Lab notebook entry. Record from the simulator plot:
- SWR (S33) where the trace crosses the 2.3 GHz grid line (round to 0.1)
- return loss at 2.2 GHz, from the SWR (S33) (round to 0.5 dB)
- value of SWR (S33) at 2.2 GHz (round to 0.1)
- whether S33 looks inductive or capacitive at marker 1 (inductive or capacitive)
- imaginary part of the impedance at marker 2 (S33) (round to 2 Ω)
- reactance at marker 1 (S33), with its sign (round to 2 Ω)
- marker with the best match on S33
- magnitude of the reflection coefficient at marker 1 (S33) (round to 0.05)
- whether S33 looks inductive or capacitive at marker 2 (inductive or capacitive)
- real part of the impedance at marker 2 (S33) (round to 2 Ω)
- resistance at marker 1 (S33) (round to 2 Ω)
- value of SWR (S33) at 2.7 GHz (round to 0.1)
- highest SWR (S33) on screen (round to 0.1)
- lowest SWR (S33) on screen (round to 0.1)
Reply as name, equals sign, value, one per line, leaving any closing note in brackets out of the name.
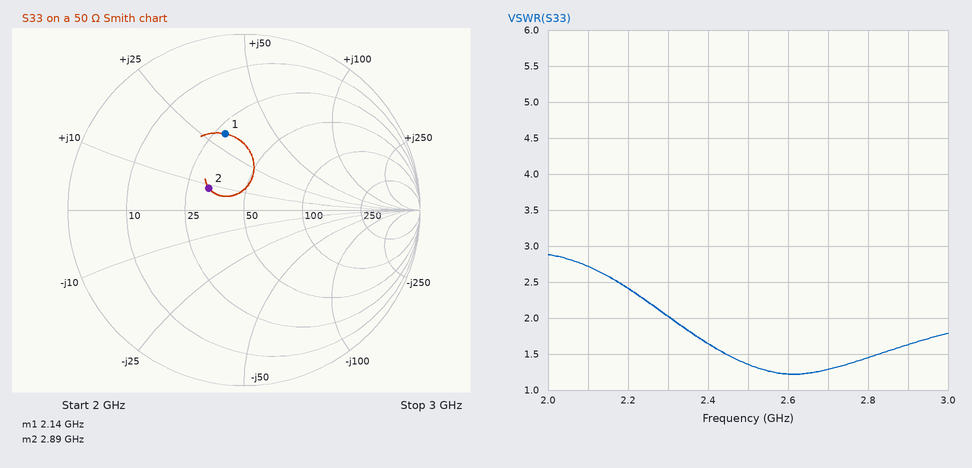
SWR (S33) where the trace crosses the 2.3 GHz grid line = 2.0
return loss at 2.2 GHz, from the SWR (S33) = 7.5 dB
value of SWR (S33) at 2.2 GHz = 2.4
whether S33 looks inductive or capacitive at marker 1 = inductive
imaginary part of the impedance at marker 2 (S33) = +8 Ω
reactance at marker 1 (S33), with its sign = +30 Ω
marker with the best match on S33 = marker 2
magnitude of the reflection coefficient at marker 1 (S33) = 0.45
whether S33 looks inductive or capacitive at marker 2 = inductive
real part of the impedance at marker 2 (S33) = 32 Ω
resistance at marker 1 (S33) = 28 Ω
value of SWR (S33) at 2.7 GHz = 1.3
highest SWR (S33) on screen = 2.9
lowest SWR (S33) on screen = 1.2
